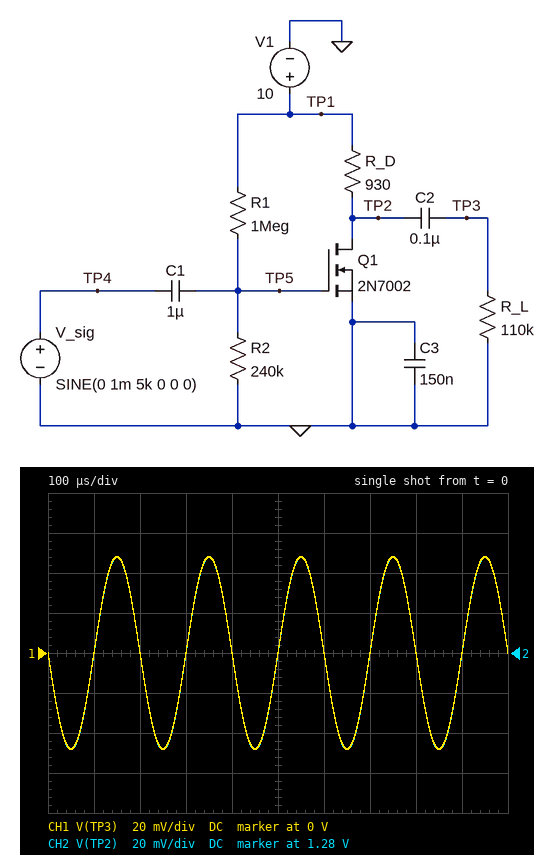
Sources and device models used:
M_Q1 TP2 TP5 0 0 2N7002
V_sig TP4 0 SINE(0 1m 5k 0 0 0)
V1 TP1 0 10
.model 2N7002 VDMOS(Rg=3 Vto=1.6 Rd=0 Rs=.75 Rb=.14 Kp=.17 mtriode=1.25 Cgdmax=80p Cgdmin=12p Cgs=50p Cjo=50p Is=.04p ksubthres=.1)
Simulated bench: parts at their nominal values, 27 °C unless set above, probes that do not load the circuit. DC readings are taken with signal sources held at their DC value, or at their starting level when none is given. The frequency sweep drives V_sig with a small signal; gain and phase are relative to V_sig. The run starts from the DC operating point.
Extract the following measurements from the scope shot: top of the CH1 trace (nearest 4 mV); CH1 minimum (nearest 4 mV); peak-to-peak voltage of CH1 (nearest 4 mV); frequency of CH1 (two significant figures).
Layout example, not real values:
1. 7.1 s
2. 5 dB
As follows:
1. 48 mV
2. -48 mV
3. 96 mV
4. 5.0 kHz
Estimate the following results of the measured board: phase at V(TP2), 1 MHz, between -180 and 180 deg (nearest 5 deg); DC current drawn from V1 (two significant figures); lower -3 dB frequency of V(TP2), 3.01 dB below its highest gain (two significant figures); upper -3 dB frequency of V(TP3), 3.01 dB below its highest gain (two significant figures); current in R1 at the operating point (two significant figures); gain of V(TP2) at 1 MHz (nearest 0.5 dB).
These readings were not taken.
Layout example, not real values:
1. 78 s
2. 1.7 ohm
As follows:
1. 145 deg
2. 9.4 mA
3. 810 mHz
4. 1.6 MHz
5. 8.1 µA
6. 32.0 dB
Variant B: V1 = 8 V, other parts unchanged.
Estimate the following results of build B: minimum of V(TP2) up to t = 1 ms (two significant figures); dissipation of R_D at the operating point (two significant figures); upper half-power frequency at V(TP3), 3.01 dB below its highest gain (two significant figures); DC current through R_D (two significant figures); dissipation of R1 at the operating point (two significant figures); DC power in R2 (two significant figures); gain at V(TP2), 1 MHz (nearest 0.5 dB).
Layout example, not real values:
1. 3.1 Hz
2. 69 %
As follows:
1. 7.8 V
2. 32 µW
3. 5.7 MHz
4. 190 µA
5. 42 µW
6. 10 µW
7. 8.5 dB
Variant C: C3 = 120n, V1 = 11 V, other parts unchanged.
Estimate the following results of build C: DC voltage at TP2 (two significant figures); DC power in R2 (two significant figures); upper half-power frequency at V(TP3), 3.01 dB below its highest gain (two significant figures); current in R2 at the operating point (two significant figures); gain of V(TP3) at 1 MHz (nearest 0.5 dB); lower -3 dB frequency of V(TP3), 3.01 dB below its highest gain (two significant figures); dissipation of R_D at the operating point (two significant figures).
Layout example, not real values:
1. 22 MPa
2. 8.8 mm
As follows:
1. 130 mV
2. 19 µW
3. 870 MHz
4. 8.9 µA
5. -9.5 dB
6. 30 MHz
7. 130 mW
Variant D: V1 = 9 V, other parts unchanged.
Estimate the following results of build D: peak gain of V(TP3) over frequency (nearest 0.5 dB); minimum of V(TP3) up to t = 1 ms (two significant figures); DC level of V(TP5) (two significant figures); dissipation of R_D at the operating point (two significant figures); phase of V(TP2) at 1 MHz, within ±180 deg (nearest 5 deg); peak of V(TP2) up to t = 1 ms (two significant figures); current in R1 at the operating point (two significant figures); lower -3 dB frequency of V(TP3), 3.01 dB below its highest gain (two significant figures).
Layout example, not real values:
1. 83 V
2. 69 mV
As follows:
1. 26.0 dB
2. -20 mV
3. 1.7 V
4. 4.7 mW
5. 170 deg
6. 6.9 V
7. 7.3 µA
8. 14 Hz
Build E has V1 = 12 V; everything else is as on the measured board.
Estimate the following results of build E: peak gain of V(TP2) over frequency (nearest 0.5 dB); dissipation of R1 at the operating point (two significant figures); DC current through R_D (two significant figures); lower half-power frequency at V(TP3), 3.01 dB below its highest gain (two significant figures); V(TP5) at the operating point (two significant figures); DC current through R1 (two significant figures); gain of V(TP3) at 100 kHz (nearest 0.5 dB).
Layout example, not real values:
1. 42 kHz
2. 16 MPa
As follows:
1. -6.5 dB
2. 94 µW
3. 13 mA
4. 84 MHz
5. 2.3 V
6. 9.7 µA
7. -16.5 dB
